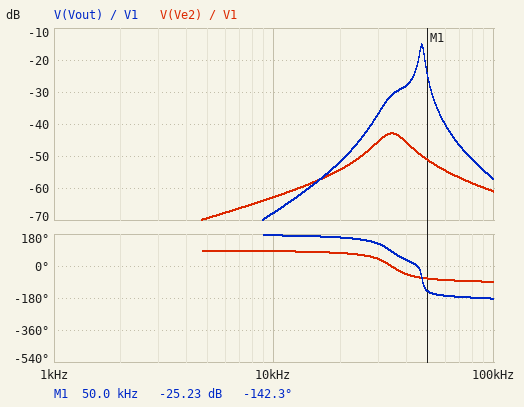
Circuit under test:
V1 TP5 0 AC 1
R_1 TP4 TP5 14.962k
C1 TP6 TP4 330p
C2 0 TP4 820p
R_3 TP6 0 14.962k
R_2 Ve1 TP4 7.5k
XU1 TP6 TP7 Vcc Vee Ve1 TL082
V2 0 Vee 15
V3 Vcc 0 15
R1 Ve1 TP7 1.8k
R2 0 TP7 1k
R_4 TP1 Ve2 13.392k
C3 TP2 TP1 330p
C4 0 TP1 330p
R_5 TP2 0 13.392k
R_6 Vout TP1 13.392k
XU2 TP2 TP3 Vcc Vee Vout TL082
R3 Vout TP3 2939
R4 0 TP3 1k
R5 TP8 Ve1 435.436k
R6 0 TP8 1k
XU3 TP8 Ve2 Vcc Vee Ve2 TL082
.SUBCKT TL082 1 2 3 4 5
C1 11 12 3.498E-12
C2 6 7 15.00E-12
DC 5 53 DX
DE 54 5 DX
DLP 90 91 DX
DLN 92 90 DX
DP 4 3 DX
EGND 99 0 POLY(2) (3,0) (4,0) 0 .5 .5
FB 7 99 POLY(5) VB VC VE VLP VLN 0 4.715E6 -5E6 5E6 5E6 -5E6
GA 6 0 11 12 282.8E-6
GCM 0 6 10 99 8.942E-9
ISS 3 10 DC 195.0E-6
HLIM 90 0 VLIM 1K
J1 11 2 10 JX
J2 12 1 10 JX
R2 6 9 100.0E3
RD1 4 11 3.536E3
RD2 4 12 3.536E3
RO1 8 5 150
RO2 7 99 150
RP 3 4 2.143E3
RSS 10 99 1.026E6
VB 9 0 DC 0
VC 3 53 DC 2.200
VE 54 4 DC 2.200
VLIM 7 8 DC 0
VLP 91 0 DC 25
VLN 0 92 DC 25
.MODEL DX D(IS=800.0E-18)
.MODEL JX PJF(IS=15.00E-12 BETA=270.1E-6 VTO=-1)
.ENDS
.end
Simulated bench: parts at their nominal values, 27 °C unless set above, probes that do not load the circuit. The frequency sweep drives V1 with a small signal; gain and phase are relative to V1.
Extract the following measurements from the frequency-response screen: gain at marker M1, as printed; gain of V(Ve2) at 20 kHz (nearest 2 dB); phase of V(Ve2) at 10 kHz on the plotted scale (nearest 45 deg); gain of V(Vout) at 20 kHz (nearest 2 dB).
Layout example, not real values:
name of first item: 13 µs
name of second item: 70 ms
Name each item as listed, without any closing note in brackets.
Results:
gain at marker M1, as printed: -25.23 dB
gain of V(Ve2) at 20 kHz: -54 dB
phase of V(Ve2) at 10 kHz on the plotted scale: 90 deg
gain of V(Vout) at 20 kHz: -52 dB
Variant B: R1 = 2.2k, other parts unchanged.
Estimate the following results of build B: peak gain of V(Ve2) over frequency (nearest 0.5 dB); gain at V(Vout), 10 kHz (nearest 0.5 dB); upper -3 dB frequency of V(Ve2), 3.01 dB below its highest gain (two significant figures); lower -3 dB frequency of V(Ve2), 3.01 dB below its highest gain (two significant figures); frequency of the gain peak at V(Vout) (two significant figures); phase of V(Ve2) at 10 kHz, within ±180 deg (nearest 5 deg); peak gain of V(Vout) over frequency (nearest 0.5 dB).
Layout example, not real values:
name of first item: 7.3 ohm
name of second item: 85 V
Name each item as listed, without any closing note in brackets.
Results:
peak gain of V(Ve2) over frequency: -23.0 dB
gain at V(Vout), 10 kHz: -66.5 dB
upper -3 dB frequency of V(Ve2), 3.01 dB below its highest gain: 35 kHz
lower -3 dB frequency of V(Ve2), 3.01 dB below its highest gain: 33 kHz
frequency of the gain peak at V(Vout): 34 kHz
phase of V(Ve2) at 10 kHz, within ±180 deg: 90 deg
peak gain of V(Vout) over frequency: -11.0 dB
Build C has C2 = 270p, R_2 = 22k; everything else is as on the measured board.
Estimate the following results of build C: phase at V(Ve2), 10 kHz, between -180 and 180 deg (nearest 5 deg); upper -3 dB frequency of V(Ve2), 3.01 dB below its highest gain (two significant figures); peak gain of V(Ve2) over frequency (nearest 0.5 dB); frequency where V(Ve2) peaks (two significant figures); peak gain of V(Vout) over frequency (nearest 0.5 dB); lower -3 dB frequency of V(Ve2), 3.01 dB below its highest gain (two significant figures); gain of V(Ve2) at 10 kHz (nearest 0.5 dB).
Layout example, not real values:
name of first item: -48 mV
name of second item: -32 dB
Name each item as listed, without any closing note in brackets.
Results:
phase at V(Ve2), 10 kHz, between -180 and 180 deg: 70 deg
upper -3 dB frequency of V(Ve2), 3.01 dB below its highest gain: 83 kHz
peak gain of V(Ve2) over frequency: -48.0 dB
frequency where V(Ve2) peaks: 45 kHz
peak gain of V(Vout) over frequency: -13.0 dB
lower -3 dB frequency of V(Ve2), 3.01 dB below its highest gain: 24 kHz
gain of V(Ve2) at 10 kHz: -58.5 dB
